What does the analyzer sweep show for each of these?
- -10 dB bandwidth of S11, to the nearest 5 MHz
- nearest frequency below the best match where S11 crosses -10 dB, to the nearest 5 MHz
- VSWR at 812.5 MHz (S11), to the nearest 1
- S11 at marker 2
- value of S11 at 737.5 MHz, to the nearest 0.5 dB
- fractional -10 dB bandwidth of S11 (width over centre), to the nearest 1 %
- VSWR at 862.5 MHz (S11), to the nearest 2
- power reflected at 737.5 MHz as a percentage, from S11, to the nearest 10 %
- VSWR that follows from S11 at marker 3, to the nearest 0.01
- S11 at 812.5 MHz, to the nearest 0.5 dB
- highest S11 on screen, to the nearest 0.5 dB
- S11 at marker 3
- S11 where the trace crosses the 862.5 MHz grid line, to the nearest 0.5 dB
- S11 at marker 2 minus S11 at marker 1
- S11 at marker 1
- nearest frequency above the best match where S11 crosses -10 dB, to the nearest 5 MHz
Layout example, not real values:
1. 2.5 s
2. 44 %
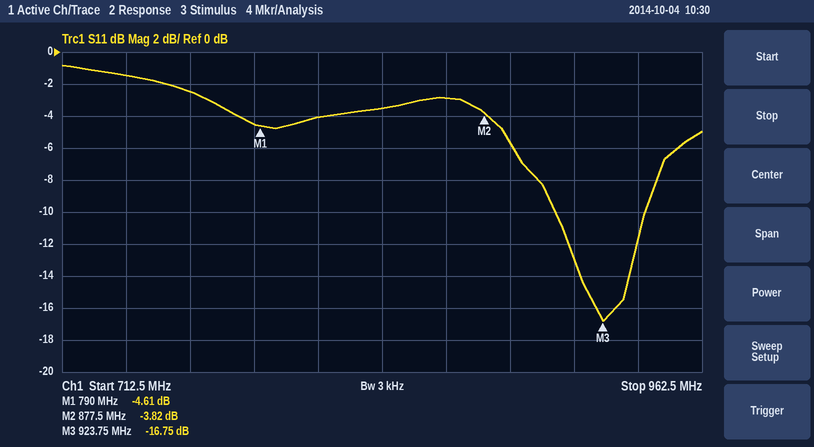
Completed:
1. 35 MHz
2. 905 MHz
3. 4
4. -3.82 dB
5. -1.5 dB
6. 4 %
7. 6
8. 70 %
9. 1.34
10. -4.0 dB
11. -1.0 dB
12. -16.75 dB
13. -3.0 dB
14. 0.79 dB
15. -4.61 dB
16. 940 MHz
